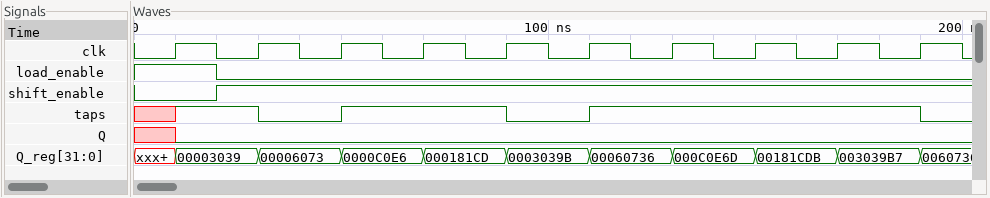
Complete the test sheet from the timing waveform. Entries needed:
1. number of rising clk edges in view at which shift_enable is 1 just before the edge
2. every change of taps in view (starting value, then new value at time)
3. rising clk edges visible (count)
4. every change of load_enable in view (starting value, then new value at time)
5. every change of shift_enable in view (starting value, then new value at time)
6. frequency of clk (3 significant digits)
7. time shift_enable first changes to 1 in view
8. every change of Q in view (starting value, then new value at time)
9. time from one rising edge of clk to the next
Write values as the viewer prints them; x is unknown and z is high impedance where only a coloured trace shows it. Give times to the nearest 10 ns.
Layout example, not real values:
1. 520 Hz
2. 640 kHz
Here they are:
1. 9
2. x, 1 at 10 ns, 0 at 30 ns, 1 at 50 ns, 0 at 90 ns, 1 at 110 ns, 0 at 190 ns
3. 10
4. 1, 0 at 20 ns
5. 0, 1 at 20 ns
6. 50.0 MHz
7. 20 ns
8. x, 0 at 10 ns
9. 20 ns
